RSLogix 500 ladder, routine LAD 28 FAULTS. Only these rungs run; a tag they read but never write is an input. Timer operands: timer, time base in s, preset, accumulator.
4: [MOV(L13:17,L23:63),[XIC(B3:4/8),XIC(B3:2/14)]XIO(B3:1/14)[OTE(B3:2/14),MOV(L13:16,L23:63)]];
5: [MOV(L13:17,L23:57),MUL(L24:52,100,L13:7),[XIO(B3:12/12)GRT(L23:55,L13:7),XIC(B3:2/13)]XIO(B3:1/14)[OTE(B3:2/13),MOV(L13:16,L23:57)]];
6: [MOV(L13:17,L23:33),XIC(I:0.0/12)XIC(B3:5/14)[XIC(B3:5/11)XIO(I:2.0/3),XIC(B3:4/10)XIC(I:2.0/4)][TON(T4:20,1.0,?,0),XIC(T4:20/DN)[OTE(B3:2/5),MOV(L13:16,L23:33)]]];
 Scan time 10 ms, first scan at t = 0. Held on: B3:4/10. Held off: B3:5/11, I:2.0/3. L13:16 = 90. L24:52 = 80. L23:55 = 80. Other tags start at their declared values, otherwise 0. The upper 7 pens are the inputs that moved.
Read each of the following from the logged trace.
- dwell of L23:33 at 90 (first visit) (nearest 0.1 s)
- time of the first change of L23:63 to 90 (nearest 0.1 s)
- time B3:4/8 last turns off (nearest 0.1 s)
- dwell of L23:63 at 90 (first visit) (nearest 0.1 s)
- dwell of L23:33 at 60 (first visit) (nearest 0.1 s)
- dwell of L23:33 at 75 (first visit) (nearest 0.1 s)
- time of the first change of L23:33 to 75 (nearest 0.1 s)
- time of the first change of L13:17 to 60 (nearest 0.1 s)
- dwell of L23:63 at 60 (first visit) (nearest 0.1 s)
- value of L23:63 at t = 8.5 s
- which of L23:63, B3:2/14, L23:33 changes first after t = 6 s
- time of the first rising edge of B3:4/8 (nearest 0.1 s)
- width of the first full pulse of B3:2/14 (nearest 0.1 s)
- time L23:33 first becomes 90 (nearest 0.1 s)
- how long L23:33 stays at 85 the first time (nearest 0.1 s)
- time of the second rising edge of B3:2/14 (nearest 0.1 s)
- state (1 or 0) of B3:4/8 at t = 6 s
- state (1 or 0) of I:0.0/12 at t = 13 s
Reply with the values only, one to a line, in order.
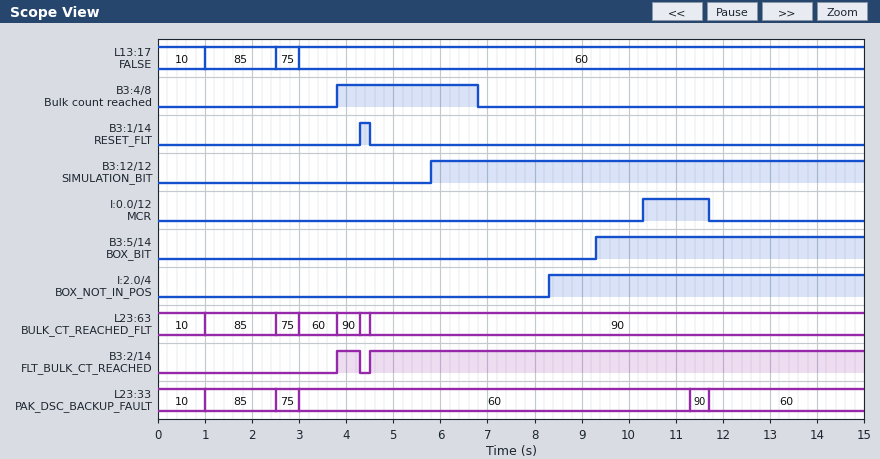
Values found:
0.4 s
3.8 s
6.8 s
0.5 s
8.3 s
0.5 s
2.5 s
3.0 s
0.8 s
90
L23:33
3.8 s
0.5 s
11.3 s
1.5 s
4.5 s
1
0
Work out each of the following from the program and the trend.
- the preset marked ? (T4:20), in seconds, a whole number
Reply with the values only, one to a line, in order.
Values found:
1 s
